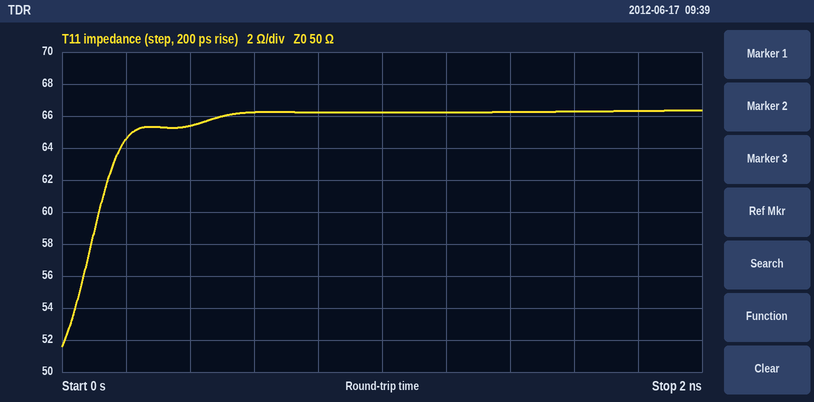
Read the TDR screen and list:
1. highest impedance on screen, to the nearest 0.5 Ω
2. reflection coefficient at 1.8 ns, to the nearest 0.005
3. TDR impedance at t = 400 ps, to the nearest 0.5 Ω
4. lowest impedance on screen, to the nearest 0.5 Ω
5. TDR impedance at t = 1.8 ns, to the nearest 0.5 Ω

66.5 Ω
+0.140
65.5 Ω
51.5 Ω
66.5 Ω
